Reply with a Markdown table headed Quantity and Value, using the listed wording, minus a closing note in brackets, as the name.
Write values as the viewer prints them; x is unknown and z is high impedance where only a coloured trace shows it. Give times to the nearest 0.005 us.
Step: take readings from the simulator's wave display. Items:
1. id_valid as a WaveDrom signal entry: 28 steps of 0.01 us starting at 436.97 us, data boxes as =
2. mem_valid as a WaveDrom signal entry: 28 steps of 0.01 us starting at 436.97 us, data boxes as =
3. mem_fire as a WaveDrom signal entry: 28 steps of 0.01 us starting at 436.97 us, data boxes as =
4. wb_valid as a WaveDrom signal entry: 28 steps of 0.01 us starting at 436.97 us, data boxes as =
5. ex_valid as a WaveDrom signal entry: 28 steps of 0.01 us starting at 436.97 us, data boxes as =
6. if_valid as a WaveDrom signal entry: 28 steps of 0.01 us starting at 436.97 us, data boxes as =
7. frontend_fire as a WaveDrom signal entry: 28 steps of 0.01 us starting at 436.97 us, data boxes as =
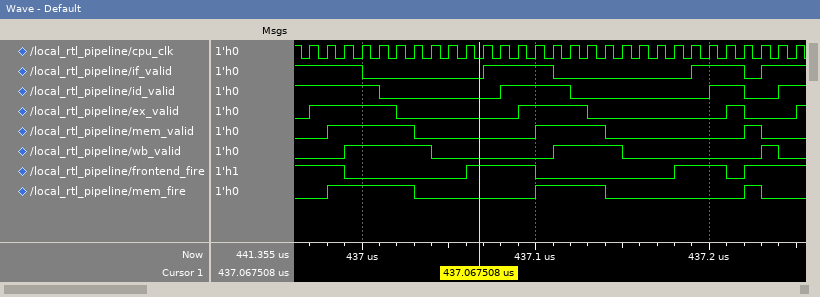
| Quantity | Value |
|---|---|
| id_valid as a WaveDrom signal entry: 28 steps of 0.01 us starting at 436.97 us, data boxes as = | {name: 'id_valid', wave: '1...0......1...0.......1.0.1'} |
| mem_valid as a WaveDrom signal entry: 28 steps of 0.01 us starting at 436.97 us, data boxes as = | {name: 'mem_valid', wave: '01....0......1...0.......10.'} |
| mem_fire as a WaveDrom signal entry: 28 steps of 0.01 us starting at 436.97 us, data boxes as = | {name: 'mem_fire', wave: '01....0......1...0.......10.'} |
| wb_valid as a WaveDrom signal entry: 28 steps of 0.01 us starting at 436.97 us, data boxes as = | {name: 'wb_valid', wave: '0.1....0......1...0.......10'} |
| ex_valid as a WaveDrom signal entry: 28 steps of 0.01 us starting at 436.97 us, data boxes as = | {name: 'ex_valid', wave: '1....0......1...0.......10..'} |
| if_valid as a WaveDrom signal entry: 28 steps of 0.01 us starting at 436.97 us, data boxes as = | {name: 'if_valid', wave: '1..0......1...0.......1..01.'} |
| frontend_fire as a WaveDrom signal entry: 28 steps of 0.01 us starting at 436.97 us, data boxes as = | {name: 'frontend_fire', wave: '1.0......1...0.......1..01..'} |
